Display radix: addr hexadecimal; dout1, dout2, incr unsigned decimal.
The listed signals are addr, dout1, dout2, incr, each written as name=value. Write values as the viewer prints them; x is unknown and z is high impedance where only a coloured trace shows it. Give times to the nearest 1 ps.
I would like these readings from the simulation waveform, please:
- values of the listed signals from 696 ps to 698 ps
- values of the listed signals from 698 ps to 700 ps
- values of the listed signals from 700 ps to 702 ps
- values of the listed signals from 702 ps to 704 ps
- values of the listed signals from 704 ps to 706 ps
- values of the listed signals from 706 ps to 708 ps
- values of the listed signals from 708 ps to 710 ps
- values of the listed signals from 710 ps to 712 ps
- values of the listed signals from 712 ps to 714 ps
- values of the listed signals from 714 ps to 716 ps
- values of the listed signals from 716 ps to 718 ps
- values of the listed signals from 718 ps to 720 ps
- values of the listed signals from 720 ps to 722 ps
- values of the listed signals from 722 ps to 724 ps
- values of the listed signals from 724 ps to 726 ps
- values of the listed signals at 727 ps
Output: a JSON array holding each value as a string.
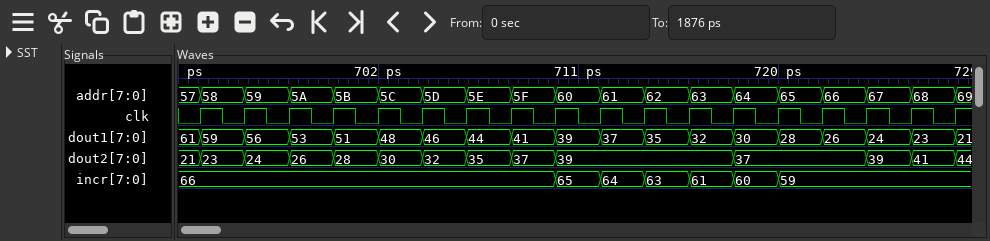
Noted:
["addr=59, dout1=56, dout2=24, incr=66", "addr=5A, dout1=53, dout2=26, incr=66", "addr=5B, dout1=51, dout2=28, incr=66", "addr=5C, dout1=48, dout2=30, incr=66", "addr=5D, dout1=46, dout2=32, incr=66", "addr=5E, dout1=44, dout2=35, incr=66", "addr=5F, dout1=41, dout2=37, incr=66", "addr=60, dout1=39, dout2=39, incr=65", "addr=61, dout1=37, dout2=39, incr=64", "addr=62, dout1=35, dout2=39, incr=63", "addr=63, dout1=32, dout2=39, incr=61", "addr=64, dout1=30, dout2=37, incr=60", "addr=65, dout1=28, dout2=37, incr=59", "addr=66, dout1=26, dout2=37, incr=59", "addr=67, dout1=24, dout2=39, incr=59", "addr=68, dout1=23, dout2=41, incr=59"]
